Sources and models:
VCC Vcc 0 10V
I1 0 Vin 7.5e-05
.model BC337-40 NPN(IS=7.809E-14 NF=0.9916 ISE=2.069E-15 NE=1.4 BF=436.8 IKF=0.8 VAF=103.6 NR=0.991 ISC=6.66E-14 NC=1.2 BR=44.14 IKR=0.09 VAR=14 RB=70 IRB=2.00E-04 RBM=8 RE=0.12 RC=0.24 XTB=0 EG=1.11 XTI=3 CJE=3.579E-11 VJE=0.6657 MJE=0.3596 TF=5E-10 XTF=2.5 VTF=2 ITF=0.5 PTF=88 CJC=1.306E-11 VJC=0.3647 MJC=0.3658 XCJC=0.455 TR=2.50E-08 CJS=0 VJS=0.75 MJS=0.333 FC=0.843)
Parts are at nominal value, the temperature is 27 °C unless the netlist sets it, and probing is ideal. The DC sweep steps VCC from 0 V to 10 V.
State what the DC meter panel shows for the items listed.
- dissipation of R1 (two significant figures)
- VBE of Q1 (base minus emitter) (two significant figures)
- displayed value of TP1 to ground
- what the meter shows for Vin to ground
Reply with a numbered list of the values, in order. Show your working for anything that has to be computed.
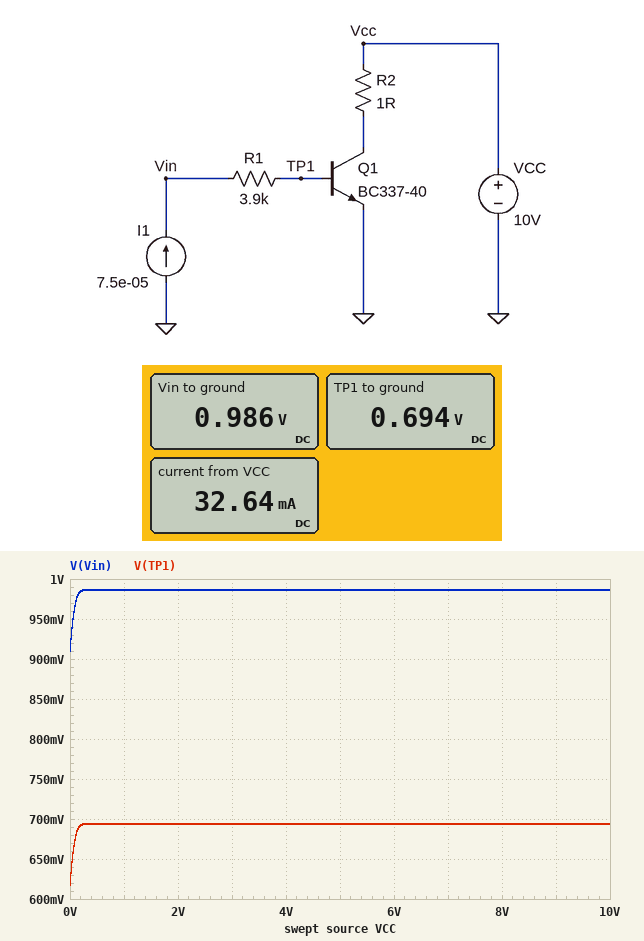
1. (986 mV - 694 mV)^2 / 3.9 kΩ = 22 µW
2. 694 mV = 690 mV
3. 0.694 V
4. 0.986 V
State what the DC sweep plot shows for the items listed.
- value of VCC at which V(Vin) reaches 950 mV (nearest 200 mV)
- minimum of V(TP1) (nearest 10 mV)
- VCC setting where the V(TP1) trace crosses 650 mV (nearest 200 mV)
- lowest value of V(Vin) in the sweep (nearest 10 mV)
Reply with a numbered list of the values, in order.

1. 0 V
2. 620 mV
3. 0 V
4. 910 mV
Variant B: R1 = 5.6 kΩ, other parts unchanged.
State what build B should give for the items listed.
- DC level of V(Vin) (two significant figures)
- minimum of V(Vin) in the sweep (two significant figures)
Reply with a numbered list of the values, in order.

1. 1.1 V
2. 1.0 V
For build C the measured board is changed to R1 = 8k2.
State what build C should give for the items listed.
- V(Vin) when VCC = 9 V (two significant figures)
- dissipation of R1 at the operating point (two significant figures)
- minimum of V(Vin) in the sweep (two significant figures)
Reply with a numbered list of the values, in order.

1. 1.3 V
2. 46 µW
3. 1.2 V
